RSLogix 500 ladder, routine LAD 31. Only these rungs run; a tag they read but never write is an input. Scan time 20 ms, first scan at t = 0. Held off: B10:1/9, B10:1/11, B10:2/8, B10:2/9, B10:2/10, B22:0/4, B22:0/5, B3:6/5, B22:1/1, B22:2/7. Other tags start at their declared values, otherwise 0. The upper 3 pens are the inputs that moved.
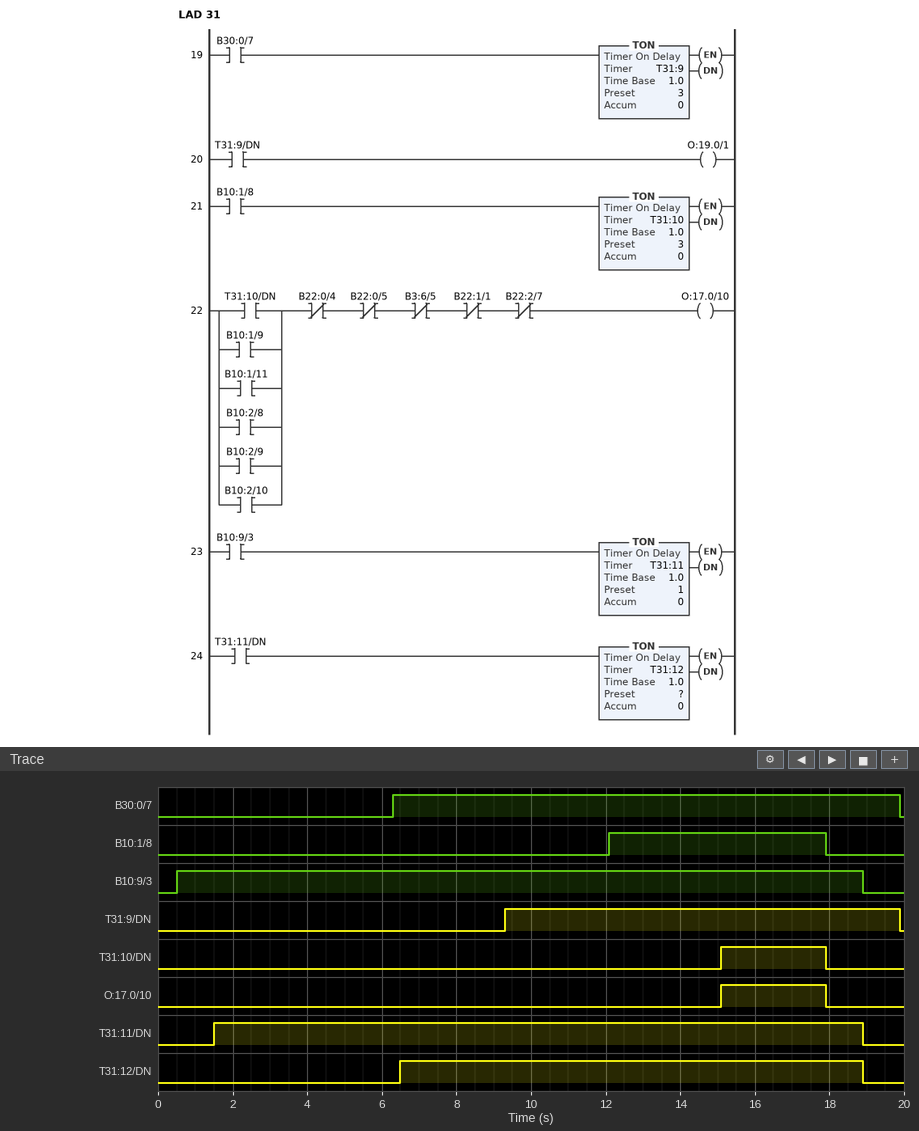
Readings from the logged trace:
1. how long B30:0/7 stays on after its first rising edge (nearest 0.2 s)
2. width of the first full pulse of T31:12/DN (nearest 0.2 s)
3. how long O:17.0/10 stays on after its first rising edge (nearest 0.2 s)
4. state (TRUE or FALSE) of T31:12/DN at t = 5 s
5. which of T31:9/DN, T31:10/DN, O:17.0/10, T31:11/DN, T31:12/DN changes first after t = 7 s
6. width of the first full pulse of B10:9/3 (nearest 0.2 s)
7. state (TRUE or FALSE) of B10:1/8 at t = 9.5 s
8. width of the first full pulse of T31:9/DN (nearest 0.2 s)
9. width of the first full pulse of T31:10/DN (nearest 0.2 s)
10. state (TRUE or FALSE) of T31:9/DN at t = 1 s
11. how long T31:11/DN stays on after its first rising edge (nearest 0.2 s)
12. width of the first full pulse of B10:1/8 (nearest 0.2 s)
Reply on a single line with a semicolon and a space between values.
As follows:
13.6 s; 12.4 s; 2.8 s; FALSE; T31:9/DN; 18.4 s; FALSE; 10.6 s; 2.8 s; FALSE; 17.4 s; 5.8 s
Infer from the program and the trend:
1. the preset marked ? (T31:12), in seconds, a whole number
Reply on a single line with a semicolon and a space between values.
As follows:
5 s
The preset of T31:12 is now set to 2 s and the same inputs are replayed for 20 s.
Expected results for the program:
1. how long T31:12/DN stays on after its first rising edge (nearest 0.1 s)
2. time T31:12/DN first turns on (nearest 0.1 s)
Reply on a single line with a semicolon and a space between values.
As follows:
15.4 s; 3.5 s
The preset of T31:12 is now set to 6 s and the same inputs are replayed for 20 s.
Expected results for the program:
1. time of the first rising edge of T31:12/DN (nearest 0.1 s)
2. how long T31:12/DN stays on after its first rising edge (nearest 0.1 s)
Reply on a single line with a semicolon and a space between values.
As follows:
7.5 s; 11.4 s
